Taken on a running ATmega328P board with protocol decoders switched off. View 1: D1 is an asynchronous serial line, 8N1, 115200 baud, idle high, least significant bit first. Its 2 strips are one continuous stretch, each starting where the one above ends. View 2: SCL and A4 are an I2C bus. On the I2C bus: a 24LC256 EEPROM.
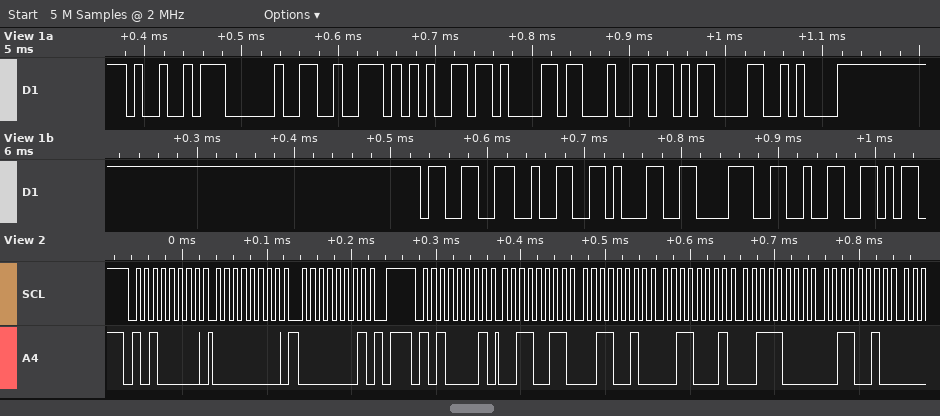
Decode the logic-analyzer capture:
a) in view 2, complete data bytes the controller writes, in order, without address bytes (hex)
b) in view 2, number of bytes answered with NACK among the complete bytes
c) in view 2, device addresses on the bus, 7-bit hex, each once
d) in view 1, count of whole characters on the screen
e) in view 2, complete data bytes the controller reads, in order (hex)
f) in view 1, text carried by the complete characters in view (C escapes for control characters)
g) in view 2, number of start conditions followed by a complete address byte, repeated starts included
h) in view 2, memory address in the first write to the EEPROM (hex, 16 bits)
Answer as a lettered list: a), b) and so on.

a) 00 01
b) 0
c) 0x50
d) 13
e) 33 32 31 38 32
f) "I read\r\n32182"
g) 2
h) 0x0001
